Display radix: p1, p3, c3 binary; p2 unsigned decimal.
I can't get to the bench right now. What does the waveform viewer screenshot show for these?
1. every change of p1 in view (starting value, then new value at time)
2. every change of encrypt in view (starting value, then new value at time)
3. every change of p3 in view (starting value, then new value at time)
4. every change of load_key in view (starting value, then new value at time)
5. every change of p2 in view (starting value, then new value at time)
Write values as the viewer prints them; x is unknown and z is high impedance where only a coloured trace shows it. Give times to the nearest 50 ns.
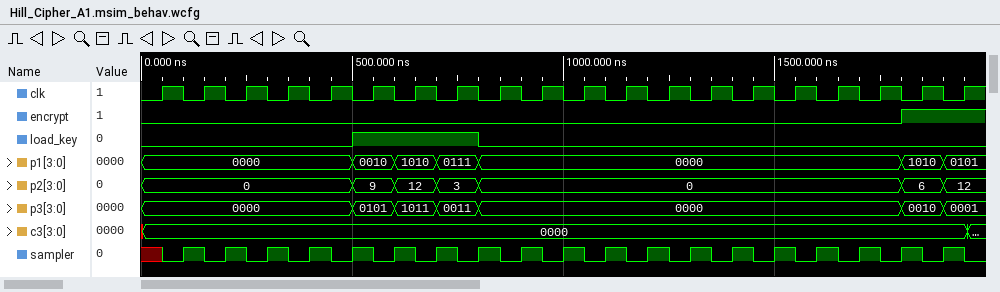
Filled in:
0000, 0010 at 500 ns, 1010 at 600 ns, 0111 at 700 ns, 0000 at 800 ns, 1010 at 1800 ns, 0101 at 1900 ns
0, 1 at 1800 ns
0000, 0101 at 500 ns, 1011 at 600 ns, 0011 at 700 ns, 0000 at 800 ns, 0010 at 1800 ns, 0001 at 1900 ns
0, 1 at 500 ns, 0 at 800 ns
0, 9 at 500 ns, 12 at 600 ns, 3 at 700 ns, 0 at 800 ns, 6 at 1800 ns, 12 at 1900 ns
